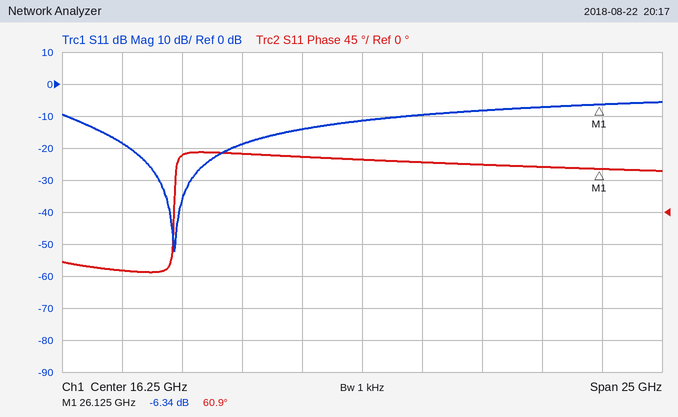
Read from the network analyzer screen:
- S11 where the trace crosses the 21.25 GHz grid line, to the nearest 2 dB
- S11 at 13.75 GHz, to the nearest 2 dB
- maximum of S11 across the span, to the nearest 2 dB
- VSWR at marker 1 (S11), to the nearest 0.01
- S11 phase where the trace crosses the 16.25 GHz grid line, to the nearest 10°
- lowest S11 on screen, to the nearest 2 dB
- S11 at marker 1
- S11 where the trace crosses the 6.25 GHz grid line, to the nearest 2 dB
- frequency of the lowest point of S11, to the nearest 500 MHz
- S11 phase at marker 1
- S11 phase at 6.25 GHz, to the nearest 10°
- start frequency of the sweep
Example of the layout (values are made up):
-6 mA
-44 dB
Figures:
-8 dB
-14 dB
-6 dB
2.86
70°
-52 dB
-6.34 dB
-18 dB
8.5 GHz
60.9°
-80°
3.75 GHz
